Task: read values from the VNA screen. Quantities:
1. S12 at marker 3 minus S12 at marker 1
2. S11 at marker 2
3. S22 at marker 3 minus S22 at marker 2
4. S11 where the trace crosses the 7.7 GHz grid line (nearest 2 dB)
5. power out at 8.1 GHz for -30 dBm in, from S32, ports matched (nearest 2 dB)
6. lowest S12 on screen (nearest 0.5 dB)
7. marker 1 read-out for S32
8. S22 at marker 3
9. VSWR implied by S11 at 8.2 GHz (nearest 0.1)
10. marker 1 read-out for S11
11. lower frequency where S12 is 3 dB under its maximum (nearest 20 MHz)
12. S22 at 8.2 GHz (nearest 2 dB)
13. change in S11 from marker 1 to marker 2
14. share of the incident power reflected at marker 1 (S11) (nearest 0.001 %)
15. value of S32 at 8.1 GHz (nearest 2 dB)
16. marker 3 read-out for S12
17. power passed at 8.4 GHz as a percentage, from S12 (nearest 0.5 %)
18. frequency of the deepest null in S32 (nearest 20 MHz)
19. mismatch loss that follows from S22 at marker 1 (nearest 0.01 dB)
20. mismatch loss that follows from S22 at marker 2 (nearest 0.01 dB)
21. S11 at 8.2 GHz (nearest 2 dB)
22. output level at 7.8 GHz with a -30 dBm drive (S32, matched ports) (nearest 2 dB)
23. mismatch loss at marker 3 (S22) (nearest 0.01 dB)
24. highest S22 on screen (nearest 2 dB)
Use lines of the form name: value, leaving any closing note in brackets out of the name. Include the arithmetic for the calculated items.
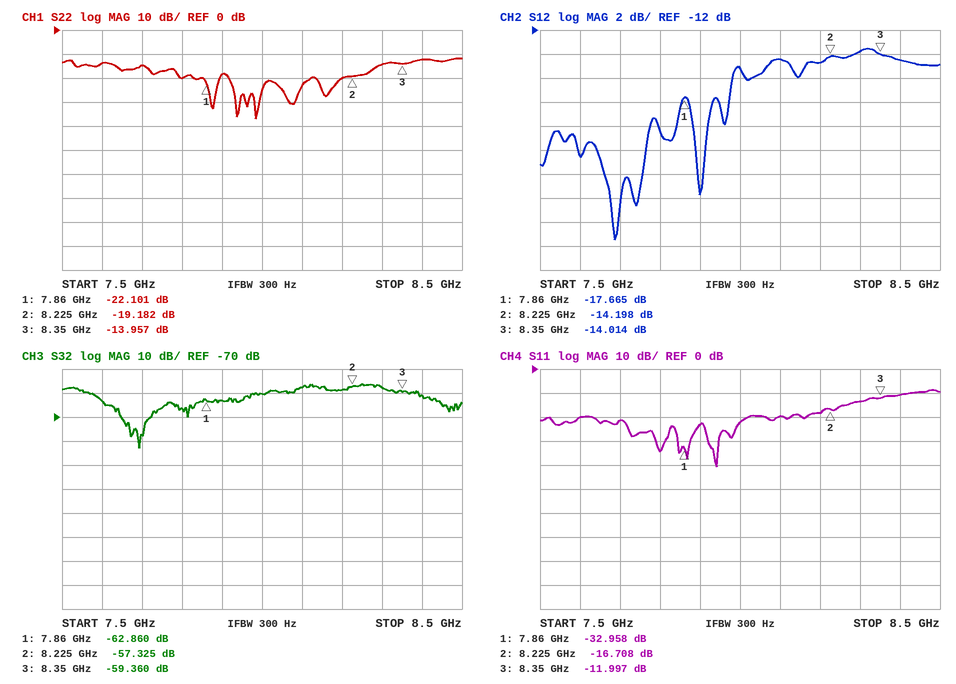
S12 at marker 3 minus S12 at marker 1: -14.014 − (-17.665) = 3.651 dB
S11 at marker 2: -16.708 dB
S22 at marker 3 minus S22 at marker 2: -13.957 − (-19.182) = 5.225 dB
S11 where the trace crosses the 7.7 GHz grid line: -22 dB
power out at 8.1 GHz for -30 dBm in, from S32, ports matched: -30 dBm + (-58 dB) = -88 dBm
lowest S12 on screen: -29.5 dB
marker 1 read-out for S32: -62.860 dB
S22 at marker 3: -13.957 dB
VSWR implied by S11 at 8.2 GHz: |Γ| = 10^(-18/20) = 0.1259; VSWR = (1 + 0.1259)/(1 − 0.1259) ≈ 1.3
marker 1 read-out for S11: -32.958 dB
lower frequency where S12 is 3 dB under its maximum: 7.98 GHz
S22 at 8.2 GHz: -20 dB
change in S11 from marker 1 to marker 2: -16.708 − (-32.958) = 16.250 dB
share of the incident power reflected at marker 1 (S11): 10^(-32.958/10) ≈ 0.051 %
value of S32 at 8.1 GHz: -58 dB
marker 3 read-out for S12: -14.014 dB
power passed at 8.4 GHz as a percentage, from S12: 10^(-14.5/10) ≈ 3.5 %
frequency of the deepest null in S32: 7.70 GHz
mismatch loss that follows from S22 at marker 1: −10 log10(1 − 10^(-22.101/10)) ≈ 0.03 dB
mismatch loss that follows from S22 at marker 2: −10 log10(1 − 10^(-19.182/10)) ≈ 0.05 dB
S11 at 8.2 GHz: -18 dB
output level at 7.8 GHz with a -30 dBm drive (S32, matched ports): -30 dBm + (-66 dB) = -96 dBm
mismatch loss at marker 3 (S22): −10 log10(1 − 10^(-13.957/10)) ≈ 0.18 dB
highest S22 on screen: -12 dB
